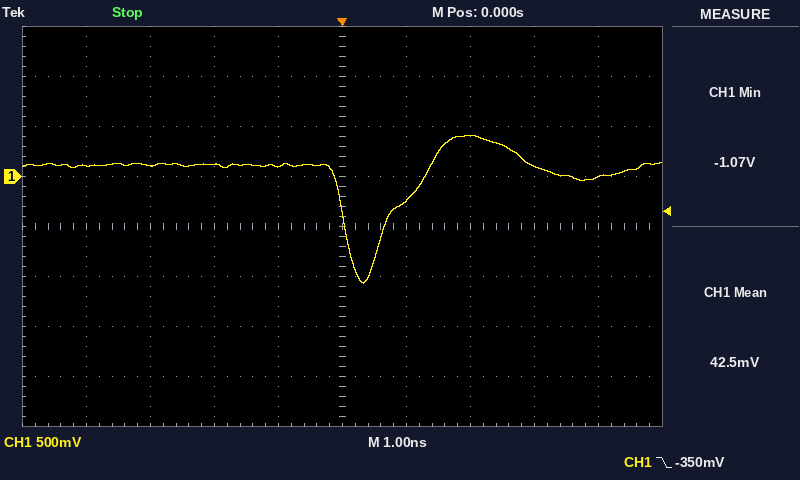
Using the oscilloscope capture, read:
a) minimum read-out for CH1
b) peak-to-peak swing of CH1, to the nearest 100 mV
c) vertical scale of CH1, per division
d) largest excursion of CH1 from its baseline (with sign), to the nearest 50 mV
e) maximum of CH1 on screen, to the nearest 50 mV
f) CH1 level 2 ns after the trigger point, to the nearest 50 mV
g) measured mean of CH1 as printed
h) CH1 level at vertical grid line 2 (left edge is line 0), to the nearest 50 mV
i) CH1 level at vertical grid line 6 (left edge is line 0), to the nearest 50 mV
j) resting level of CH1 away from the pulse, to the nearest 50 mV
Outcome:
-1.07 V
1.50 V
500 mV
-1.20 V
400 mV
400 mV
42.5 mV
100 mV
-250 mV
100 mV
